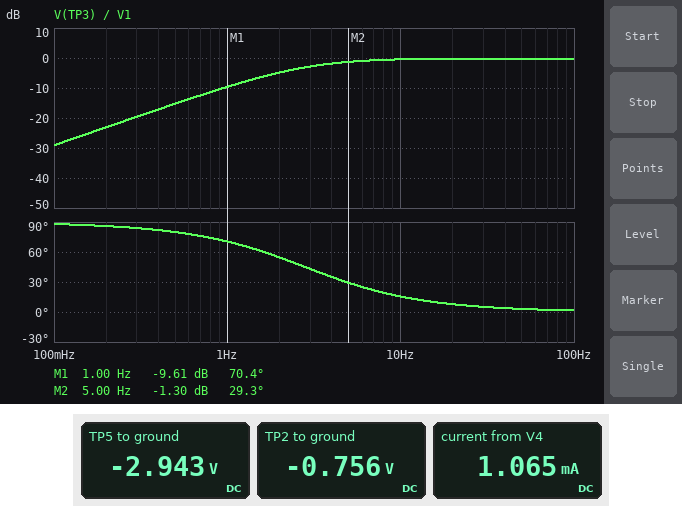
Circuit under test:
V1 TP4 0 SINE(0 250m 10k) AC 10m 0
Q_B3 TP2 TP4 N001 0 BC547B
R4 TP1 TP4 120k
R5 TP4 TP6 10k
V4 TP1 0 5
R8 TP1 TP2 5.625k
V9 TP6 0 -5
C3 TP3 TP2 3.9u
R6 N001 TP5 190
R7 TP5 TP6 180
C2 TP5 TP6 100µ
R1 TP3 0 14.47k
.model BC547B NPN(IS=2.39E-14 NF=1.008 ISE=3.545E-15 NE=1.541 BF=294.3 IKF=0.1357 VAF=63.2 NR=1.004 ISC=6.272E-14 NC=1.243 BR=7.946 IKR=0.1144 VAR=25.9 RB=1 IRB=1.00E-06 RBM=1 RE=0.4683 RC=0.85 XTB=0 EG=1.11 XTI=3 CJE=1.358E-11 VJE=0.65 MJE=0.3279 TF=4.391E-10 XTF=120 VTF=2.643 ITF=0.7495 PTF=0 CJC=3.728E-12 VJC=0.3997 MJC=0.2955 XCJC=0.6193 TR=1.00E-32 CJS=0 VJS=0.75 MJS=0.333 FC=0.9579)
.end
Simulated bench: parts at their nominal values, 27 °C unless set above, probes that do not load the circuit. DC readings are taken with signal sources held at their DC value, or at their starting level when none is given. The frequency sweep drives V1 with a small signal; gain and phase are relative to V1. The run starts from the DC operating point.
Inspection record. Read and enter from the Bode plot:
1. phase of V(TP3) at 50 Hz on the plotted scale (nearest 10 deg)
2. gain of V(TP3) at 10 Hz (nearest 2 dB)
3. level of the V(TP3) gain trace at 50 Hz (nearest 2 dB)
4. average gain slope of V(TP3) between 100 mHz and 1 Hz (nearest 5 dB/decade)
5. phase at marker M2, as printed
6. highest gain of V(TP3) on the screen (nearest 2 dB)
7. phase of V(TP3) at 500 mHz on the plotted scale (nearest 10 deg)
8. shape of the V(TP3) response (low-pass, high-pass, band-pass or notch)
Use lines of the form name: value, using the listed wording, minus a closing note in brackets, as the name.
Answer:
phase of V(TP3) at 50 Hz on the plotted scale: 0 deg
gain of V(TP3) at 10 Hz: 0 dB
level of the V(TP3) gain trace at 50 Hz: 0 dB
average gain slope of V(TP3) between 100 mHz and 1 Hz: 20 dB/decade
phase at marker M2, as printed: 29.3 deg
highest gain of V(TP3) on the screen: 0 dB
phase of V(TP3) at 500 mHz on the plotted scale: 80 deg
shape of the V(TP3) response: high-pass
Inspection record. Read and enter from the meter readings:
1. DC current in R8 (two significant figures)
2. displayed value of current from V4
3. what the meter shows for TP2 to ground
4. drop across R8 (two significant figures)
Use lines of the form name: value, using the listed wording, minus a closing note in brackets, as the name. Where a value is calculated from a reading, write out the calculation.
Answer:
DC current in R8: (5 V - (-756 mV)) / 5.625 kΩ = 1.0 mA
displayed value of current from V4: 1.065 mA
what the meter shows for TP2 to ground: -0.756 V
drop across R8: 5 V - (-756 mV) = 5.8 V
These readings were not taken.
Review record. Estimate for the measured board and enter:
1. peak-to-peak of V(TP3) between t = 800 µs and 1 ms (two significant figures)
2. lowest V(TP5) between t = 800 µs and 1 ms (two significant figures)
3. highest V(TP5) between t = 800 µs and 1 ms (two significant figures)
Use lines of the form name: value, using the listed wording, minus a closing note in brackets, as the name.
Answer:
peak-to-peak of V(TP3) between t = 800 µs and 1 ms: 490 mV
lowest V(TP5) between t = 800 µs and 1 ms: -2.9 V
highest V(TP5) between t = 800 µs and 1 ms: -2.9 V
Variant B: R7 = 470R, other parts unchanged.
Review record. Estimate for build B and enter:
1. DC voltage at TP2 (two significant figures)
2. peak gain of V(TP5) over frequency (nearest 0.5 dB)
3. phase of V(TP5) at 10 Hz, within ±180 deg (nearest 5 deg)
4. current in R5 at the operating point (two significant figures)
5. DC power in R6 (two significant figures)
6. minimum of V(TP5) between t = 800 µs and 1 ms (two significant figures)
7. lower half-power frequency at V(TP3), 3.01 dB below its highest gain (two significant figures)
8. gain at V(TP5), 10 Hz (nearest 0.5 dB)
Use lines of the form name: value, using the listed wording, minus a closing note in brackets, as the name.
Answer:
DC voltage at TP2: -730 mV
peak gain of V(TP5) over frequency: -3.0 dB
phase of V(TP5) at 10 Hz, within ±180 deg: -40 deg
current in R5 at the operating point: 500 µA
DC power in R6: 7.9 mW
minimum of V(TP5) between t = 800 µs and 1 ms: -2.0 V
lower half-power frequency at V(TP3), 3.01 dB below its highest gain: 2.7 Hz
gain at V(TP5), 10 Hz: -5.5 dB
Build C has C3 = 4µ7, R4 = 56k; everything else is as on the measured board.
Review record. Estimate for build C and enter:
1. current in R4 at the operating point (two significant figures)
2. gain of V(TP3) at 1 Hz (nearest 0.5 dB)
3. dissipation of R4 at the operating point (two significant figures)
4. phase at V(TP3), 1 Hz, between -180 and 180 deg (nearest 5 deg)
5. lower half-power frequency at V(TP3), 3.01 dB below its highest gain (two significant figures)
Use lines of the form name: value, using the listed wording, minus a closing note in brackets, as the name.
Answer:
current in R4 at the operating point: 89 µA
gain of V(TP3) at 1 Hz: -8.0 dB
dissipation of R4 at the operating point: 450 µW
phase at V(TP3), 1 Hz, between -180 and 180 deg: 65 deg
lower half-power frequency at V(TP3), 3.01 dB below its highest gain: 2.3 Hz
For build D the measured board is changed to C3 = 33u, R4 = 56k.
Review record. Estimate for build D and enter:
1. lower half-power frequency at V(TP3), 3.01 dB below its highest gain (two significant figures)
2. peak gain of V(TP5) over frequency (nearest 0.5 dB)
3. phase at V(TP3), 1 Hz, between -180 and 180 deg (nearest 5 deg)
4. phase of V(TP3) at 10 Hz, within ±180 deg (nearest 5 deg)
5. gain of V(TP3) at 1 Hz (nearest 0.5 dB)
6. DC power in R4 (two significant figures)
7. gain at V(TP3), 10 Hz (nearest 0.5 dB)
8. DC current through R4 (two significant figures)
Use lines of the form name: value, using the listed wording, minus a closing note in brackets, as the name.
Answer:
lower half-power frequency at V(TP3), 3.01 dB below its highest gain: 330 mHz
peak gain of V(TP5) over frequency: -6.5 dB
phase at V(TP3), 1 Hz, between -180 and 180 deg: 20 deg
phase of V(TP3) at 10 Hz, within ±180 deg: 0 deg
gain of V(TP3) at 1 Hz: -0.5 dB
DC power in R4: 450 µW
gain at V(TP3), 10 Hz: 0 dB
DC current through R4: 89 µA
